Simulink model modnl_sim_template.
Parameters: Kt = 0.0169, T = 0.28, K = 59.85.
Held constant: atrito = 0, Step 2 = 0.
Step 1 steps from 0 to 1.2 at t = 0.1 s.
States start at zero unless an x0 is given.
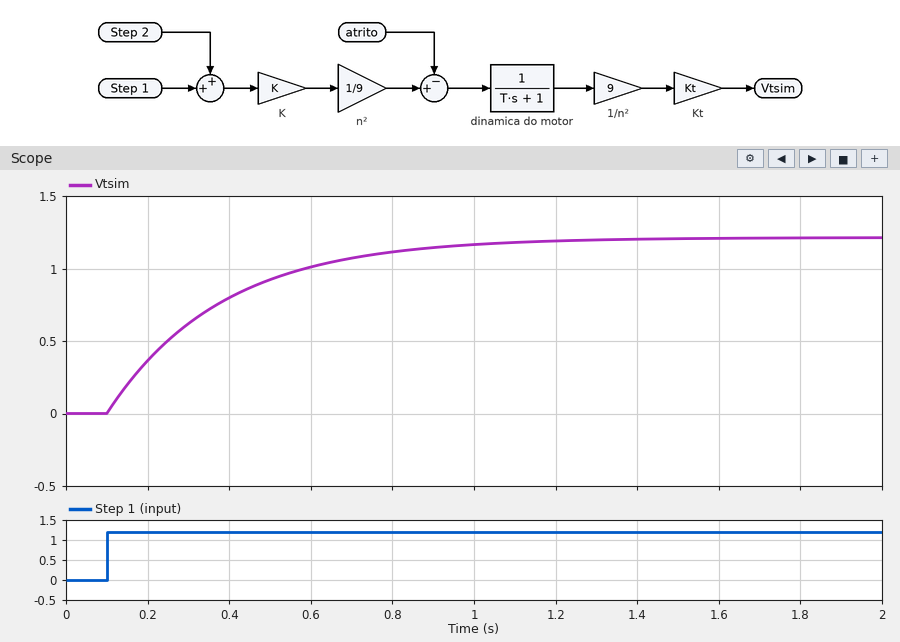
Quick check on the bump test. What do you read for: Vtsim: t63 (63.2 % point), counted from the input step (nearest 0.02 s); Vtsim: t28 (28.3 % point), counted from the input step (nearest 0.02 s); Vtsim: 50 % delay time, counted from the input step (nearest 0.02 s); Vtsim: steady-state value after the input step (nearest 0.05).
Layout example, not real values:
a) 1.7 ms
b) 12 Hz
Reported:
a) 0.28 s
b) 0.10 s
c) 0.20 s
d) 1.20
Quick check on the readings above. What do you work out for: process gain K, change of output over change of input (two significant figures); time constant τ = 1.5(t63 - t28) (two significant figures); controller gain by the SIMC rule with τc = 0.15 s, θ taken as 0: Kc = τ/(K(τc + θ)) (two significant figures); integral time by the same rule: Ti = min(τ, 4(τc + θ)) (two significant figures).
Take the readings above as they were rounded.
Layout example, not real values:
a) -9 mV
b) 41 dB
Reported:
a) 1.0
b) 0.27 s
c) 1.8
d) 0.27 s
